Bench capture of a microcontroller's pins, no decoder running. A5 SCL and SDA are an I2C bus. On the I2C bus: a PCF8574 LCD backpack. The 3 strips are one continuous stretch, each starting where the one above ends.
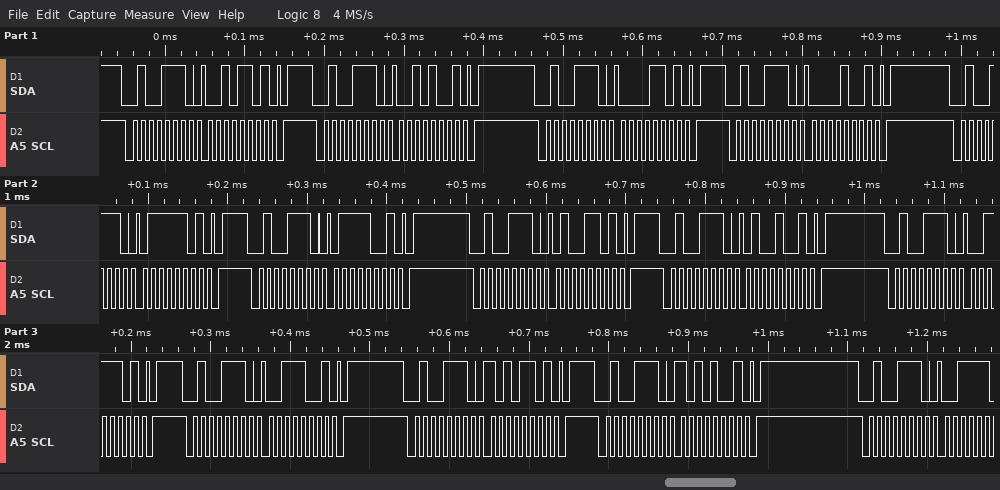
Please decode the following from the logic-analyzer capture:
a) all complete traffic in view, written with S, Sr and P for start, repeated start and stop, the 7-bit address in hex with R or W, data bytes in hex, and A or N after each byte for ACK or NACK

S 27W A 2D A P S 27W A 29 A P S 27W A 0D A P S 27W A 09 A P S 27W A 7D A P S 27W A 79 A P S 27W A 4D A P S 27W A 49 A P S 27W A 3D A P S 27W A 39 A P S 27W A AD A P S 27W A A9 A P S 27W A
